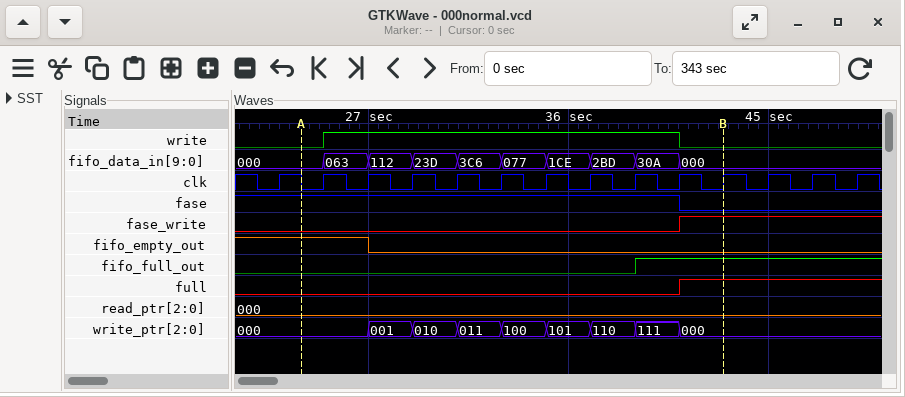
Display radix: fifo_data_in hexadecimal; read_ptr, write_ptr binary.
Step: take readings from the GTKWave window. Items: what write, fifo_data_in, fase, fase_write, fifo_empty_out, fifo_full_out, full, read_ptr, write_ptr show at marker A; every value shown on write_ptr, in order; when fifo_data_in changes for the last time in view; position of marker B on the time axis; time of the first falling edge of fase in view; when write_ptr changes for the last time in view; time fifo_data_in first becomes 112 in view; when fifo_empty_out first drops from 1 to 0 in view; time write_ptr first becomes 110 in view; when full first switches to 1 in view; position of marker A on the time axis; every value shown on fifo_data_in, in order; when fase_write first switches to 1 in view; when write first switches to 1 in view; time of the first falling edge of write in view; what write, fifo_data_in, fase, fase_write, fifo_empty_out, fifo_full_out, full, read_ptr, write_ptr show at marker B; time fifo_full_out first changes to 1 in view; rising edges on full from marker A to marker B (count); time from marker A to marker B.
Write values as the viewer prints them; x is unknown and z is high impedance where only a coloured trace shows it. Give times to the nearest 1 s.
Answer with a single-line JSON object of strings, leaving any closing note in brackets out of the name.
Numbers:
{"what write, fifo_data_in, fase, fase_write, fifo_empty_out, fifo_full_out, full, read_ptr, write_ptr show at marker A": "write=0, fifo_data_in=000, fase=1, fase_write=0, fifo_empty_out=1, fifo_full_out=0, full=0, read_ptr=000, write_ptr=000", "every value shown on write_ptr, in order": "000, 001, 010, 011, 100, 101, 110, 111, 000", "when fifo_data_in changes for the last time in view": "41 s", "position of marker B on the time axis": "43 s", "time of the first falling edge of fase in view": "41 s", "when write_ptr changes for the last time in view": "41 s", "time fifo_data_in first becomes 112 in view": "27 s", "when fifo_empty_out first drops from 1 to 0 in view": "27 s", "time write_ptr first becomes 110 in view": "37 s", "when full first switches to 1 in view": "41 s", "position of marker A on the time axis": "24 s", "every value shown on fifo_data_in, in order": "000, 063, 112, 23D, 3C6, 077, 1CE, 2BD, 30A, 000", "when fase_write first switches to 1 in view": "41 s", "when write first switches to 1 in view": "25 s", "time of the first falling edge of write in view": "41 s", "what write, fifo_data_in, fase, fase_write, fifo_empty_out, fifo_full_out, full, read_ptr, write_ptr show at marker B": "write=0, fifo_data_in=000, fase=0, fase_write=1, fifo_empty_out=0, fifo_full_out=1, full=1, read_ptr=000, write_ptr=000", "time fifo_full_out first changes to 1 in view": "39 s", "rising edges on full from marker A to marker B": "1", "time from marker A to marker B": "19 s"}
